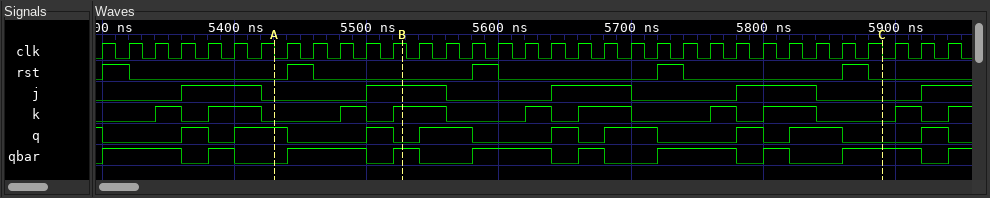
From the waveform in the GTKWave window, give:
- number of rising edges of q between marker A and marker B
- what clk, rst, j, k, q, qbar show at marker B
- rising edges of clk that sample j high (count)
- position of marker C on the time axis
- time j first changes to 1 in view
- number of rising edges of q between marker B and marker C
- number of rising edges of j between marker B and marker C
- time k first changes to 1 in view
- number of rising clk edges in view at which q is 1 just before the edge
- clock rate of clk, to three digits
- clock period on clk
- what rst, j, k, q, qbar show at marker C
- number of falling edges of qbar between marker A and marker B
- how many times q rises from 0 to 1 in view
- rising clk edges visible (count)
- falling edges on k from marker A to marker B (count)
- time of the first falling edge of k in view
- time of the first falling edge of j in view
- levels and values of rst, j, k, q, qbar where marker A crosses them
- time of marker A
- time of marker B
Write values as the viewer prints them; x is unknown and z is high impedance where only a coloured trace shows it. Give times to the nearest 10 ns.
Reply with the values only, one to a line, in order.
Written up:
1
clk=1, rst=0, j=1, k=1, q=0, qbar=1
13
5890 ns
5360 ns
5
2
5340 ns
14
50.0 MHz
20 ns
rst=0, j=0, k=0, q=0, qbar=1
1
9
33
1
5360 ns
5420 ns
rst=0, j=0, k=0, q=1, qbar=0
5430 ns
5530 ns
